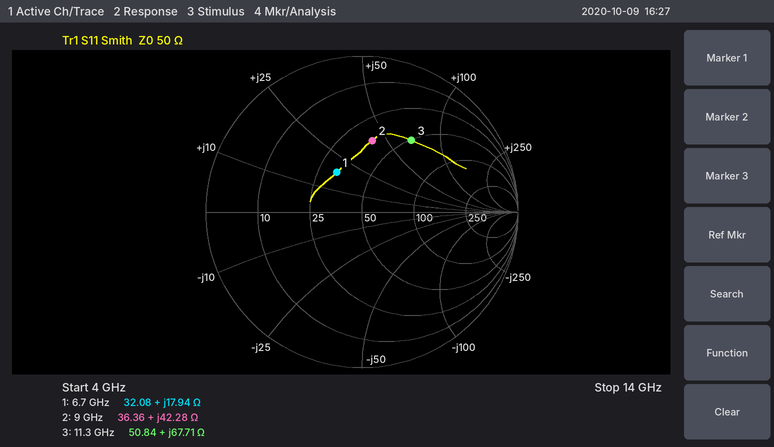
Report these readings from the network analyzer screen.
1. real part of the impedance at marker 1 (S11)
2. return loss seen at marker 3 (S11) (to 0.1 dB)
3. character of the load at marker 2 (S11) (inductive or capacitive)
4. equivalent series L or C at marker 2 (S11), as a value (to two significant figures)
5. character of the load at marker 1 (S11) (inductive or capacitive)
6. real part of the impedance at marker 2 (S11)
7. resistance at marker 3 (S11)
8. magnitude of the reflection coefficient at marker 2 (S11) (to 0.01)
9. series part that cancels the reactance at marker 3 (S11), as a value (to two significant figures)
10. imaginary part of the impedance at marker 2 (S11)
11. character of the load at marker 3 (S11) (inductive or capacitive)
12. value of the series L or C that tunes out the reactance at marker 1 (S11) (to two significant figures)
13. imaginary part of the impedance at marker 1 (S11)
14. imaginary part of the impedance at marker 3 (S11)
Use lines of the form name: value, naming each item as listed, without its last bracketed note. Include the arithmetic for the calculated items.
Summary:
real part of the impedance at marker 1: 32.08 Ω
return loss seen at marker 3 (S11): 5.1 dB
character of the load at marker 2 (S11): inductive
equivalent series L or C at marker 2 (S11), as a value: L = 42.28 Ω/(2π × 9 GHz) ≈ 748 pH, so 750 pH to two significant figures
character of the load at marker 1 (S11): inductive
real part of the impedance at marker 2: 36.36 Ω
resistance at marker 3: 50.84 Ω
magnitude of the reflection coefficient at marker 2 (S11): 0.46
series part that cancels the reactance at marker 3 (S11), as a value: C = 1/(2π × 11.3 GHz × 67.71 Ω) ≈ 208 fF, so 210 fF to two significant figures
imaginary part of the impedance at marker 2: +42.28 Ω
character of the load at marker 3 (S11): inductive
value of the series L or C that tunes out the reactance at marker 1 (S11): C = 1/(2π × 6.7 GHz × 17.94 Ω) ≈ 1.3 pF
imaginary part of the impedance at marker 1: +17.94 Ω
imaginary part of the impedance at marker 3: +67.71 Ω
